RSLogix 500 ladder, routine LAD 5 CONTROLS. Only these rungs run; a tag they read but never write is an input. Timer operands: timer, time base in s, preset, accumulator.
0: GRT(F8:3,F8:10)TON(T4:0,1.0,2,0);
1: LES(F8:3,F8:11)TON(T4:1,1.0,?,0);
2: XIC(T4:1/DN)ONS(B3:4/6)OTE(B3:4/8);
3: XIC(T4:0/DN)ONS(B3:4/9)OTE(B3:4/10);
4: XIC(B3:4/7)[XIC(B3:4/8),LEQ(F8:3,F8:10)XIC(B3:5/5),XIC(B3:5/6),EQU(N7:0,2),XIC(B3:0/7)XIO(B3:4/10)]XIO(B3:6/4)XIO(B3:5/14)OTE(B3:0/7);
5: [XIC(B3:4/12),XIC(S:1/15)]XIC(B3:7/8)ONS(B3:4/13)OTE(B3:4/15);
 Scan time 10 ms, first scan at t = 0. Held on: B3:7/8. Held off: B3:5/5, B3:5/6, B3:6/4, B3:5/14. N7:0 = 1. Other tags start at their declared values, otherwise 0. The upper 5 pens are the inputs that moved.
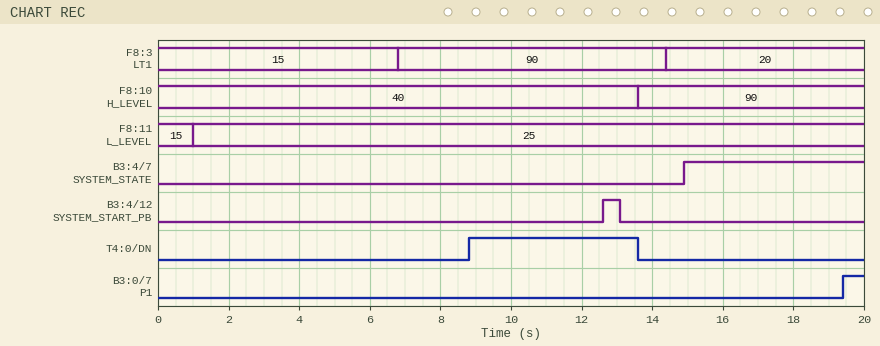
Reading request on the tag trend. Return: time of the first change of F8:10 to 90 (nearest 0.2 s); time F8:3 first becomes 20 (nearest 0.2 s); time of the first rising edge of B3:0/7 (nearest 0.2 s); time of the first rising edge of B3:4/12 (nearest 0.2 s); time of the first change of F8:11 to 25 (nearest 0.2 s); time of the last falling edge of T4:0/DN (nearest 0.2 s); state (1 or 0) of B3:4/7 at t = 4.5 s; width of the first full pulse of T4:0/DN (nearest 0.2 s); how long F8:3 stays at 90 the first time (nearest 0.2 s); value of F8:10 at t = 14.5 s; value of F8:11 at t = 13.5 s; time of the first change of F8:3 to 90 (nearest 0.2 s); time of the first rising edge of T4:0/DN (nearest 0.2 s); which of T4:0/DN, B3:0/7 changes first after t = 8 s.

13.6 s
14.4 s
19.4 s
12.6 s
1.0 s
13.6 s
0
4.8 s
7.6 s
90
25
6.8 s
8.8 s
T4:0/DN
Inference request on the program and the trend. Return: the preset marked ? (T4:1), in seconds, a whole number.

5 s
